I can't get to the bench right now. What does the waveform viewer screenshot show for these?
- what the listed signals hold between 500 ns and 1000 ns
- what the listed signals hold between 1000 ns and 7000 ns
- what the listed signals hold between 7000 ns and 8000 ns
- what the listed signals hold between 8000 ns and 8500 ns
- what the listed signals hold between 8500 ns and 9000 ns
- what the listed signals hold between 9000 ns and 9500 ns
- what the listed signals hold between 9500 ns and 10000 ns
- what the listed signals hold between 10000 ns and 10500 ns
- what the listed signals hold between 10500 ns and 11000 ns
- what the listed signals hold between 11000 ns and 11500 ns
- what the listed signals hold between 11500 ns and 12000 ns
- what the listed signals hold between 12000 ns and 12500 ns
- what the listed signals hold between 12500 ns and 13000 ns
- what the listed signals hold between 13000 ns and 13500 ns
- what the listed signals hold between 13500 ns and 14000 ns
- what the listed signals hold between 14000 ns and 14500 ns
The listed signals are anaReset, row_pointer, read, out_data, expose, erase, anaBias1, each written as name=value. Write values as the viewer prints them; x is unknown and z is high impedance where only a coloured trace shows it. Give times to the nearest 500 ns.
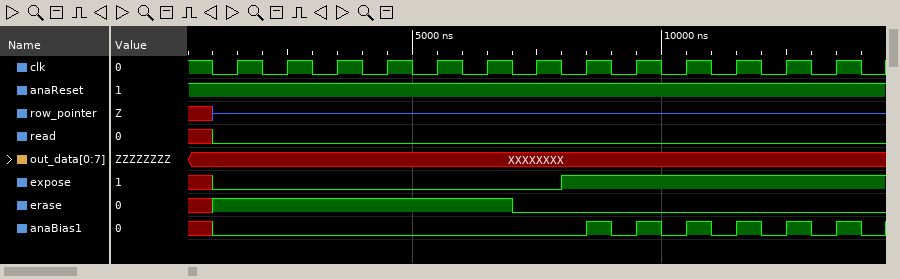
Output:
anaReset=1, row_pointer=x, read=x, out_data=XXXXXXXX, expose=x, erase=x, anaBias1=x
anaReset=1, row_pointer=z, read=0, out_data=XXXXXXXX, expose=0, erase=1, anaBias1=0
anaReset=1, row_pointer=z, read=0, out_data=XXXXXXXX, expose=0, erase=0, anaBias1=0
anaReset=1, row_pointer=z, read=0, out_data=XXXXXXXX, expose=1, erase=0, anaBias1=0
anaReset=1, row_pointer=z, read=0, out_data=XXXXXXXX, expose=1, erase=0, anaBias1=1
anaReset=1, row_pointer=z, read=0, out_data=XXXXXXXX, expose=1, erase=0, anaBias1=0
anaReset=1, row_pointer=z, read=0, out_data=XXXXXXXX, expose=1, erase=0, anaBias1=1
anaReset=1, row_pointer=z, read=0, out_data=XXXXXXXX, expose=1, erase=0, anaBias1=0
anaReset=1, row_pointer=z, read=0, out_data=XXXXXXXX, expose=1, erase=0, anaBias1=1
anaReset=1, row_pointer=z, read=0, out_data=XXXXXXXX, expose=1, erase=0, anaBias1=0
anaReset=1, row_pointer=z, read=0, out_data=XXXXXXXX, expose=1, erase=0, anaBias1=1
anaReset=1, row_pointer=z, read=0, out_data=XXXXXXXX, expose=1, erase=0, anaBias1=0
anaReset=1, row_pointer=z, read=0, out_data=XXXXXXXX, expose=1, erase=0, anaBias1=1
anaReset=1, row_pointer=z, read=0, out_data=XXXXXXXX, expose=1, erase=0, anaBias1=0
anaReset=1, row_pointer=z, read=0, out_data=XXXXXXXX, expose=1, erase=0, anaBias1=1
anaReset=1, row_pointer=z, read=0, out_data=XXXXXXXX, expose=1, erase=0, anaBias1=0
